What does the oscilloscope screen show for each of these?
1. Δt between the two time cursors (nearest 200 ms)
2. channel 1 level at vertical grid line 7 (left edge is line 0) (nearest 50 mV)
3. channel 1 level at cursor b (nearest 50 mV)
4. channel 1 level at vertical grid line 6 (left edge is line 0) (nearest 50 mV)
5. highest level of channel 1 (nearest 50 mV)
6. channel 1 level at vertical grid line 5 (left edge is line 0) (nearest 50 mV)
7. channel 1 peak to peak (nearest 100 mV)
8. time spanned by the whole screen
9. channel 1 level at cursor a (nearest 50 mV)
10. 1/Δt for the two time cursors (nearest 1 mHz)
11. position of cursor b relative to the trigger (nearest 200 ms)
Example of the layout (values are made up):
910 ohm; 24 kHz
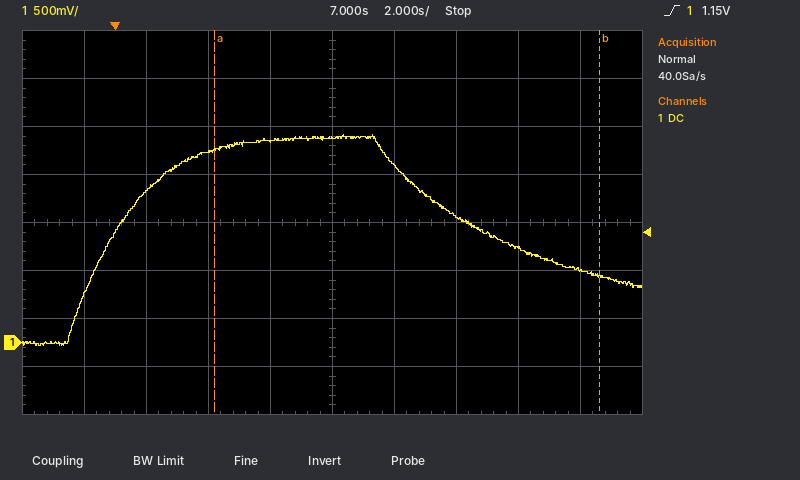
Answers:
12.4 s; 1.30 V; 700 mV; 1.85 V; 2.15 V; 2.15 V; 2.20 V; 20 s; 2.00 V; 81 mHz; +15.6 s
